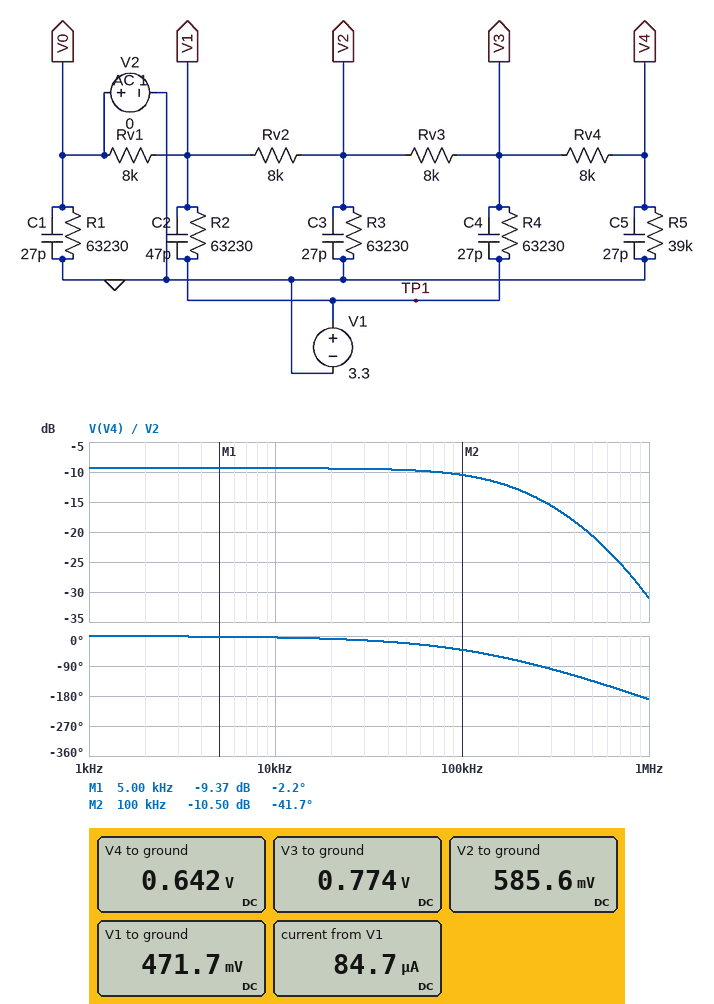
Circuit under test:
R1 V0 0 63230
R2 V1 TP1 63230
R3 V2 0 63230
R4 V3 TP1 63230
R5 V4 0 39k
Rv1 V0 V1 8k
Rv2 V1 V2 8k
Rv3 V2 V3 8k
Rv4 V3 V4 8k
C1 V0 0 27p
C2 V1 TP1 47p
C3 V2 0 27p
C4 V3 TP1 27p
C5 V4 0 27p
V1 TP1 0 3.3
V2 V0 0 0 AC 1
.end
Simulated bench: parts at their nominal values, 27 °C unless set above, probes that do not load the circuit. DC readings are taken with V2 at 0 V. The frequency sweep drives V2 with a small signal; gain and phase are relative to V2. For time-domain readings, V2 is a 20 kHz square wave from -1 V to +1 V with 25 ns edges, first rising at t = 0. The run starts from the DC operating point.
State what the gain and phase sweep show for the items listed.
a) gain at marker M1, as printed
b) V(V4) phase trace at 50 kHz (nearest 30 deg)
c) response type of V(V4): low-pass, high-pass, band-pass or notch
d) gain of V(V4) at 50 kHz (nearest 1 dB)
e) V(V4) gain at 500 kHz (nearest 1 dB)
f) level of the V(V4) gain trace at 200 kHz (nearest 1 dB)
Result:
-9.37 dB
-30 deg
low-pass
-10 dB
-21 dB
-13 dB
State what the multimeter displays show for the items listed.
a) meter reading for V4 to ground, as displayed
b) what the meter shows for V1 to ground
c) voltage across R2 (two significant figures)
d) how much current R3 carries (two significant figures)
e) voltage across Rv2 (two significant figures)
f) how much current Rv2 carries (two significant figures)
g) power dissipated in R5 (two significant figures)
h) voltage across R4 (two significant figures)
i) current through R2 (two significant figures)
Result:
0.642 V
471.7 mV
2.8 V
9.3 µA
110 mV
14 µA
11 µW
2.5 V
45 µA
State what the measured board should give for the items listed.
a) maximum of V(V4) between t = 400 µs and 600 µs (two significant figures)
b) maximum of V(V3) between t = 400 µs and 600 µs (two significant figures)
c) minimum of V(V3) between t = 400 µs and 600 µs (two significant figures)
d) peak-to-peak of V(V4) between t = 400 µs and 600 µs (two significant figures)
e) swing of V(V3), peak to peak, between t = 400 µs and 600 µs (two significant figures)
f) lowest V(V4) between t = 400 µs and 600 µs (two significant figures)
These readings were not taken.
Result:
980 mV
1.2 V
360 mV
680 mV
820 mV
300 mV
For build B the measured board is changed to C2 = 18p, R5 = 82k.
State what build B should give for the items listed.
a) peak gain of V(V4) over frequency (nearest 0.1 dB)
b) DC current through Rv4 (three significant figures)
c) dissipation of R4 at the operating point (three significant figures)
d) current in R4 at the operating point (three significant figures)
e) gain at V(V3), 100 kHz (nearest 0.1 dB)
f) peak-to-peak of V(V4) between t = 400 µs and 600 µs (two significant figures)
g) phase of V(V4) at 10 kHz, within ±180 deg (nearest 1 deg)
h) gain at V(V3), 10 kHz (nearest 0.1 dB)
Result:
-7.5 dB
9.74 µA
92.9 µW
38.3 µA
-7.9 dB
850 mV
-4 deg
-6.7 dB
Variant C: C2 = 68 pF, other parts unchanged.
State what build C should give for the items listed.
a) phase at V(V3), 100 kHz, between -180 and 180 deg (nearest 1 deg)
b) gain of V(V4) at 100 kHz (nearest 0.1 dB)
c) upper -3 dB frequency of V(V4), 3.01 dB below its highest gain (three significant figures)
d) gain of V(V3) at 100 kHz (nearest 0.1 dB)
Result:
-39 deg
-10.7 dB
164 kHz
-9.0 dB
